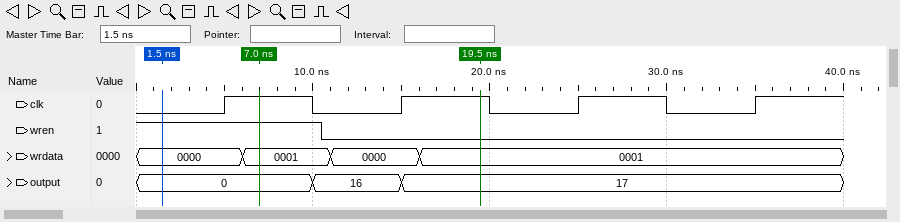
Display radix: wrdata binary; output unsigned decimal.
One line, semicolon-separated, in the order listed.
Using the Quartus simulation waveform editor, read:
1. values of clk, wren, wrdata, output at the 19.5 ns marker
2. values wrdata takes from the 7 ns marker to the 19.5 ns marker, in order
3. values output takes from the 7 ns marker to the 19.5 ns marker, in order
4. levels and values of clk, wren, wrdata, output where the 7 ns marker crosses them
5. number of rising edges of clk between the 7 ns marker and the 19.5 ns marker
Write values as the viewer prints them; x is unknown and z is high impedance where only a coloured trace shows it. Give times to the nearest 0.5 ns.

clk=1, wren=0, wrdata=0001, output=17; 0001, 0000, 0001; 0, 16, 17; clk=1, wren=1, wrdata=0001, output=0; 1
